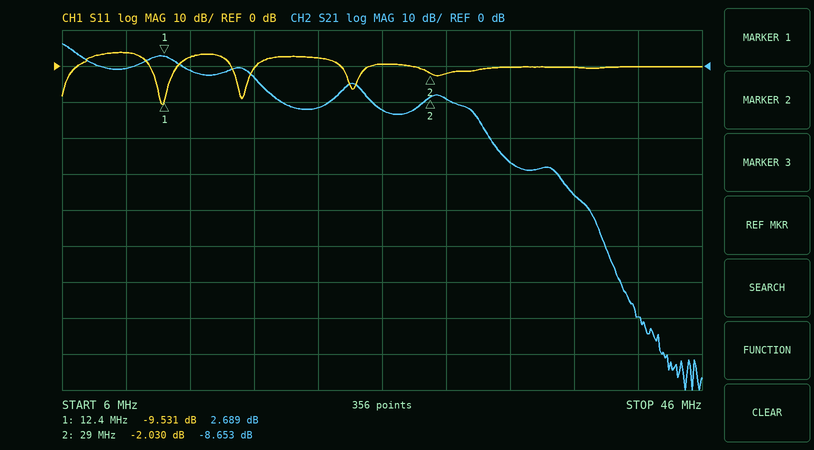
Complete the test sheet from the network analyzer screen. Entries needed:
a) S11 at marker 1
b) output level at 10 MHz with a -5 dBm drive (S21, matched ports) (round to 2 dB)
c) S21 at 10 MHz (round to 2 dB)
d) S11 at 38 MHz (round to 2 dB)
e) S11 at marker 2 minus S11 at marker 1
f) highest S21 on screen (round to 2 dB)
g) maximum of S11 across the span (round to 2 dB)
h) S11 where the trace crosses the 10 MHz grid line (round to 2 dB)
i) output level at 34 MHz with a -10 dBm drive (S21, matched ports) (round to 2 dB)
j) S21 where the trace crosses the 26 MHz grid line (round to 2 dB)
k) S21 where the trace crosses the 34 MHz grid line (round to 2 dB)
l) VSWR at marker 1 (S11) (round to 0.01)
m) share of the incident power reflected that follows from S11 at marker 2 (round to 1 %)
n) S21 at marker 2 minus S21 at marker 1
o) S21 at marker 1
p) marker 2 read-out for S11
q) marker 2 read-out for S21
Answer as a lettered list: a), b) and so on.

a) -9.531 dB
b) -6 dBm
c) 0 dB
d) 0 dB
e) 7.501 dB
f) 6 dB
g) 4 dB
h) 4 dB
i) -36 dBm
j) -12 dB
k) -26 dB
l) 2.00
m) 63 %
n) -11.342 dB
o) 2.689 dB
p) -2.030 dB
q) -8.653 dB
